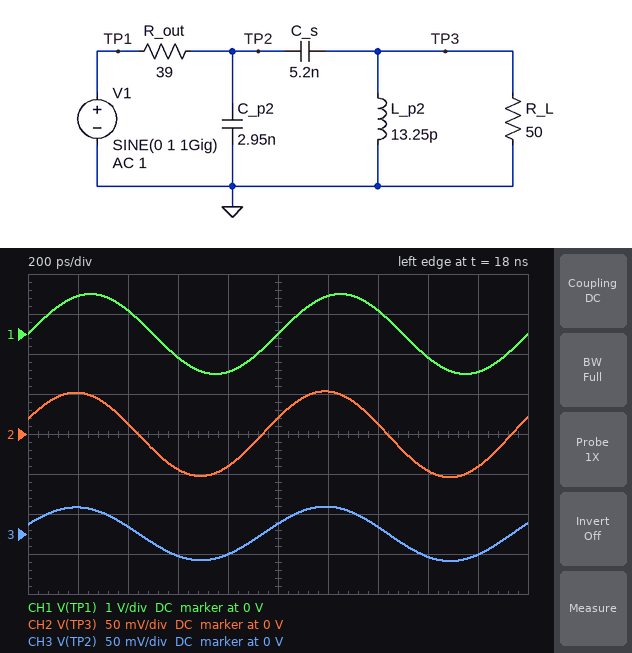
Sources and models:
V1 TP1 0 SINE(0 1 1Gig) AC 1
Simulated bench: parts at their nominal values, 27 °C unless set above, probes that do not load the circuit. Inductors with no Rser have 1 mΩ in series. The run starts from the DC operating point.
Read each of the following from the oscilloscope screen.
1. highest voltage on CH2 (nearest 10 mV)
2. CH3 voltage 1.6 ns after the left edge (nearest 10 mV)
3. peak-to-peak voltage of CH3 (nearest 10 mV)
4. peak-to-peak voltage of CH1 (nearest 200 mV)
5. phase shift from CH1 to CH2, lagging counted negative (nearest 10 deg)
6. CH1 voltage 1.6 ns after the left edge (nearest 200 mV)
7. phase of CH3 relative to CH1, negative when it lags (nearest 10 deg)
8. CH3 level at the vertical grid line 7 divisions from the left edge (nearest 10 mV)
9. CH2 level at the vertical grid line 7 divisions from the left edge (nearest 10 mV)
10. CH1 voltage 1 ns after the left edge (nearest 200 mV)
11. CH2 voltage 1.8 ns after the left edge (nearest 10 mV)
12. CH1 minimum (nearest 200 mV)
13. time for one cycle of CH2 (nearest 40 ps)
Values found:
50 mV
-30 mV
70 mV
2.0 V
20 deg
-600 mV
20 deg
10 mV
10 mV
0 V
-40 mV
-1.0 V
1.00 ns
